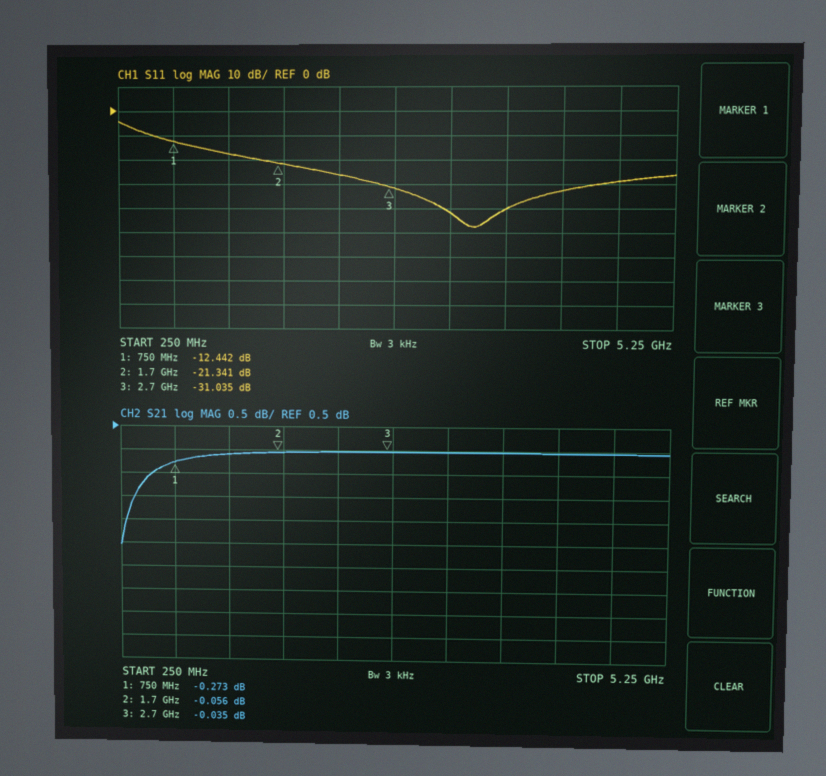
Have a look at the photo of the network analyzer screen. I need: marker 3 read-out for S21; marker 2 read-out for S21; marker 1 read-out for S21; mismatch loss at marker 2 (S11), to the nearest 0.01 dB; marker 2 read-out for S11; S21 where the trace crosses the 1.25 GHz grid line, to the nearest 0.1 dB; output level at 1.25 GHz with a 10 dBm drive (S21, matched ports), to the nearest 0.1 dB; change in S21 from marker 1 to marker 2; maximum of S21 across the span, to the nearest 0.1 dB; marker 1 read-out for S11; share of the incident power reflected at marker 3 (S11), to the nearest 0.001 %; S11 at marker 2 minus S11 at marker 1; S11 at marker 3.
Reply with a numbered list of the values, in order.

1. -0.035 dB
2. -0.056 dB
3. -0.273 dB
4. 0.03 dB
5. -21.341 dB
6. -0.1 dB
7. 9.9 dBm
8. 0.217 dB
9. 0.0 dB
10. -12.442 dB
11. 0.079 %
12. -8.899 dB
13. -31.035 dB
